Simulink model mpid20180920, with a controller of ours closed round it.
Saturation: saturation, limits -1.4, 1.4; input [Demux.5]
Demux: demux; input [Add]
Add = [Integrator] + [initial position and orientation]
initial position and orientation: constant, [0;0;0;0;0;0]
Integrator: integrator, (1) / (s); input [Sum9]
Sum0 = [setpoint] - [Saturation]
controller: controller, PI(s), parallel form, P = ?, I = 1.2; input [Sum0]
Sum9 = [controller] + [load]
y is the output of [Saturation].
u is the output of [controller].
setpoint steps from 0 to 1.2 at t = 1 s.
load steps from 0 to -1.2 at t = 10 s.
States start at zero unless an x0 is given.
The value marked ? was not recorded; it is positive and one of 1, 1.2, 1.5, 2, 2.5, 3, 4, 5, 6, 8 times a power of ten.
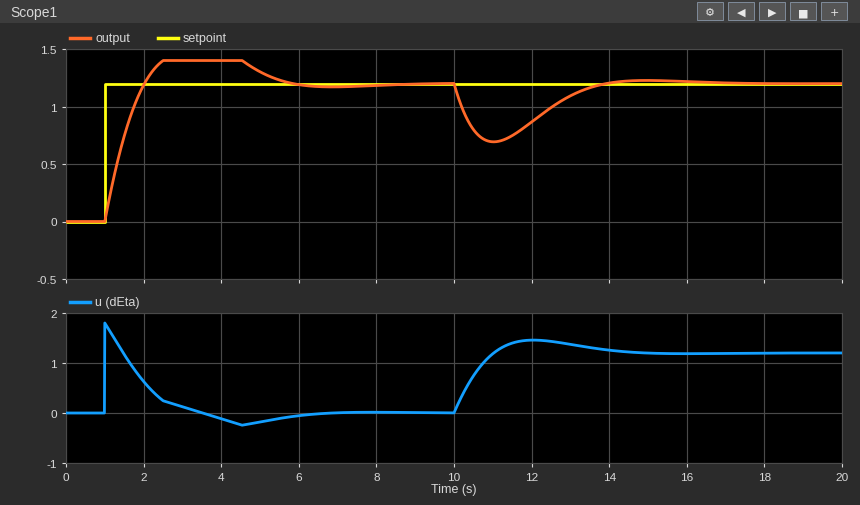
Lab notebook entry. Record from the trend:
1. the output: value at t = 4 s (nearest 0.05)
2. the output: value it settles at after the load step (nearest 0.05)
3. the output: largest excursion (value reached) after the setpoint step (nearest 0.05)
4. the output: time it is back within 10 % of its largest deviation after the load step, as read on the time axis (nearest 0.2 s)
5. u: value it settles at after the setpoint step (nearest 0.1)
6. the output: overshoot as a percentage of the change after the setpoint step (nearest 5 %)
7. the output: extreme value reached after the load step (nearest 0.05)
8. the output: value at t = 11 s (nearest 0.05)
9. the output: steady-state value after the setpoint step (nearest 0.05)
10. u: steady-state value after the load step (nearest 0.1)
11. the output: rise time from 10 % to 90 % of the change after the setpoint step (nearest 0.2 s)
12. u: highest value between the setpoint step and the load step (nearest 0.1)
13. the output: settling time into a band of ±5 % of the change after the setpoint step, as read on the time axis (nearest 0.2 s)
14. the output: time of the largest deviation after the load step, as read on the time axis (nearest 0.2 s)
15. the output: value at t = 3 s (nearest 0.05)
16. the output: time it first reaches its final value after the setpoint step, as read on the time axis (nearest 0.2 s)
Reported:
1.40
1.20
1.40
13.4 s
0.0
15 %
0.70
0.70
1.20
1.2
0.8 s
1.8
5.2 s
11.0 s
1.40
2.0 s
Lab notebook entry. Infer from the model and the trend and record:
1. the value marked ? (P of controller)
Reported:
1.5
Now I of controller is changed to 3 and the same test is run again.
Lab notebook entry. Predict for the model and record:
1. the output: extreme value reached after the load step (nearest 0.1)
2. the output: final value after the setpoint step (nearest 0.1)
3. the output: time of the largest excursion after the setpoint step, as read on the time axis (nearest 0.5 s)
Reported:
0.8
1.2
2.0 s
